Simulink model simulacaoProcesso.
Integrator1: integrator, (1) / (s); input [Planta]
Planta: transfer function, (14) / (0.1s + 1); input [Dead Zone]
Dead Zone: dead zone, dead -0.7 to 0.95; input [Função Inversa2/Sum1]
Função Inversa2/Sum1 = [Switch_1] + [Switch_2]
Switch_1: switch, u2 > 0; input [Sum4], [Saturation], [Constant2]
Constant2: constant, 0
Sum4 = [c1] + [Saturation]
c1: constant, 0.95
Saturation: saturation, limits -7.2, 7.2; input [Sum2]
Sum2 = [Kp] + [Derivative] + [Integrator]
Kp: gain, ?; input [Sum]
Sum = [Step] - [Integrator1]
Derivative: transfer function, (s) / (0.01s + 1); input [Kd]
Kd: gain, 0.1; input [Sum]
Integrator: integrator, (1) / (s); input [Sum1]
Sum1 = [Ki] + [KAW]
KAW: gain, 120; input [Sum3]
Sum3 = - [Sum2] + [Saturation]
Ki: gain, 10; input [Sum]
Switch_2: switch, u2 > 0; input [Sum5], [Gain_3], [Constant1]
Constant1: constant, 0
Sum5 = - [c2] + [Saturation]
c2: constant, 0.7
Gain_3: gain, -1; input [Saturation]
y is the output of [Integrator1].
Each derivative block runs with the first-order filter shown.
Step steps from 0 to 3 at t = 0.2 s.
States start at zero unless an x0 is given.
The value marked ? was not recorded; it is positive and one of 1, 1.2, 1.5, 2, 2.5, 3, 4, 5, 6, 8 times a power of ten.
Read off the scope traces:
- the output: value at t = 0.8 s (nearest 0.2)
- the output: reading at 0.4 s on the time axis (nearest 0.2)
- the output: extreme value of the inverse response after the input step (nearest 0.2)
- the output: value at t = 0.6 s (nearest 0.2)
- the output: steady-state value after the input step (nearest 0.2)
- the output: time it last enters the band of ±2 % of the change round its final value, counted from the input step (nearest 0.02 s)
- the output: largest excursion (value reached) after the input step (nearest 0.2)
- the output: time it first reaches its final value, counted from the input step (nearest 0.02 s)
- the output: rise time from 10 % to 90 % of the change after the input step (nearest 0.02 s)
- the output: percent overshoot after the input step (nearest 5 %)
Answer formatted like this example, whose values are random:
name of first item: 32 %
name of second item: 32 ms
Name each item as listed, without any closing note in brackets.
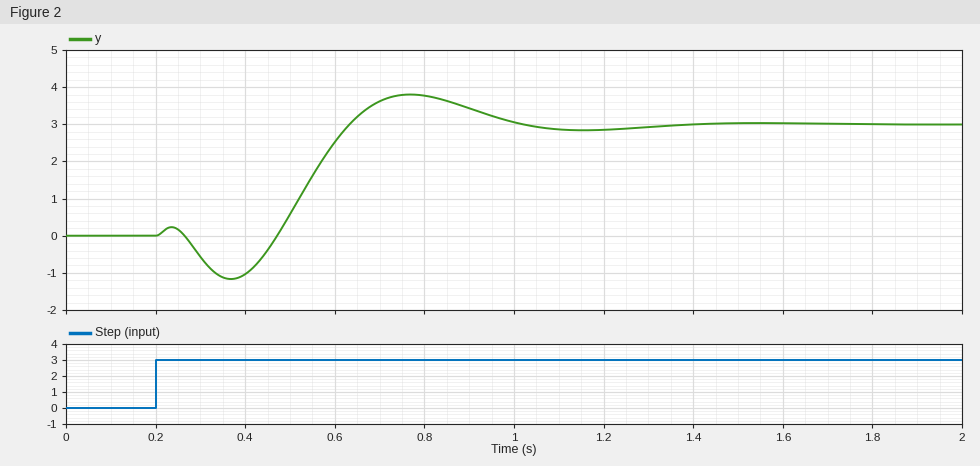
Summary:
the output: value at t = 0.8 s: 3.8
the output: reading at 0.4 s on the time axis: -1.0
the output: extreme value of the inverse response after the input step: -1.2
the output: value at t = 0.6 s: 2.6
the output: steady-state value after the input step: 3.0
the output: time it last enters the band of ±2 % of the change round its final value, counted from the input step: 1.12 s
the output: largest excursion (value reached) after the input step: 3.8
the output: time it first reaches its final value, counted from the input step: 0.44 s
the output: rise time from 10 % to 90 % of the change after the input step: 0.12 s
the output: percent overshoot after the input step: 25 %
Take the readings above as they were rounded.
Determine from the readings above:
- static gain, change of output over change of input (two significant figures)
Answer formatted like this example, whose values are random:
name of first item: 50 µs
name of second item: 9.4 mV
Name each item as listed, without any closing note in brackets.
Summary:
static gain, change of output over change of input: 1.0
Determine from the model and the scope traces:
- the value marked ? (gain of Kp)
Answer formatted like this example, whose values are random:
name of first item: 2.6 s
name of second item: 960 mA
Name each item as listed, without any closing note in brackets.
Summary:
the value marked ?: 1.5
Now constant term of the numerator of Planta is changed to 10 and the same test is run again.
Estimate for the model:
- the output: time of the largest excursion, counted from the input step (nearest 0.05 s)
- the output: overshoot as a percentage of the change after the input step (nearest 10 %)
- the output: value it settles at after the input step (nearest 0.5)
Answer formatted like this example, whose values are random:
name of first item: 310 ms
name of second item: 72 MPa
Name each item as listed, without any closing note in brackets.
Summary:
the output: time of the largest excursion, counted from the input step: 0.60 s
the output: overshoot as a percentage of the change after the input step: 40 %
the output: value it settles at after the input step: 3.0
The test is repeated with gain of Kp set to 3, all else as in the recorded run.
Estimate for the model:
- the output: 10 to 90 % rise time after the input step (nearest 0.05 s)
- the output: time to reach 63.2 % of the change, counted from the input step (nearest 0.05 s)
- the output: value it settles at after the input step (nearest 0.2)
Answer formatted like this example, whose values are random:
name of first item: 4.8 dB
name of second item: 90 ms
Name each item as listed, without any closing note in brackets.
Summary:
the output: 10 to 90 % rise time after the input step: 0.70 s
the output: time to reach 63.2 % of the change, counted from the input step: 0.40 s
the output: value it settles at after the input step: 3.0
